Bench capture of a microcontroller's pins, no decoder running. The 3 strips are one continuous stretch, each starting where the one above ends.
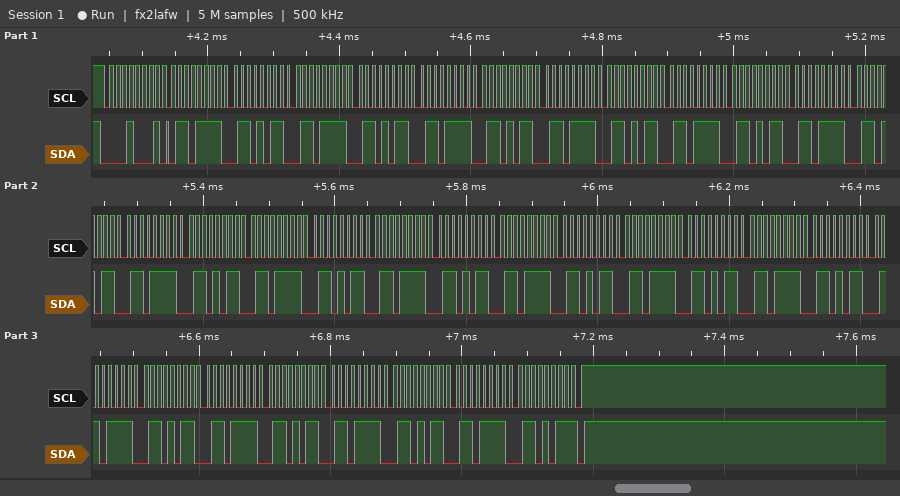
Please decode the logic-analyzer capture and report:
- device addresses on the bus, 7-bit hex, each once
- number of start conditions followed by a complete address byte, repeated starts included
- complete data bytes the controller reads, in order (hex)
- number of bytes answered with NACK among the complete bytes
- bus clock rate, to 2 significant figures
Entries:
0x08
1
6F 6B 6F 6B 6F 6B 6F 6B 6F 6B 6F 6B 6F 6B 6F 6B 6F 6B 6F 6B 6F 6B 6F 6B 6F 6B 6F 6B 6F 6B 6F 6B
1
100 kHz
